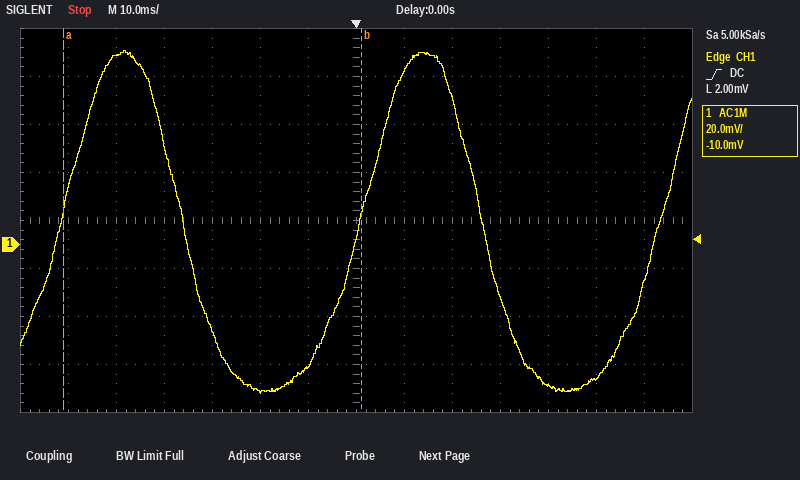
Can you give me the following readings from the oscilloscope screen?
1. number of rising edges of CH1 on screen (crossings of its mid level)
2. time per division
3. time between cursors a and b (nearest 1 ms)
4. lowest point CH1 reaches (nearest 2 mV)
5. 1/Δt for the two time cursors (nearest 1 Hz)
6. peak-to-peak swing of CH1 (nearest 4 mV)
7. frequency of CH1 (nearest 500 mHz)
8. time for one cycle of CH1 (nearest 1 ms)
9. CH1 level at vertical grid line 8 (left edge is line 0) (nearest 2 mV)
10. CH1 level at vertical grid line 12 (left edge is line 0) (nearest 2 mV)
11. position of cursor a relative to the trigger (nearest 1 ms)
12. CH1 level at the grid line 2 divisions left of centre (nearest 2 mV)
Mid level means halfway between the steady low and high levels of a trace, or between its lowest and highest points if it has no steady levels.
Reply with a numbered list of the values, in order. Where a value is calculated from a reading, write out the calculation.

1. 3
2. 10 ms
3. 62 ms
4. -62 mV
5. 1 / 62 ms ≈ 16 Hz
6. 144 mV
7. 1 / 62 ms ≈ 16.1 Hz, so 16.0 Hz to the nearest 500 mHz
8. 62 ms
9. 72 mV
10. -56 mV
11. -61 ms
12. -62 mV
